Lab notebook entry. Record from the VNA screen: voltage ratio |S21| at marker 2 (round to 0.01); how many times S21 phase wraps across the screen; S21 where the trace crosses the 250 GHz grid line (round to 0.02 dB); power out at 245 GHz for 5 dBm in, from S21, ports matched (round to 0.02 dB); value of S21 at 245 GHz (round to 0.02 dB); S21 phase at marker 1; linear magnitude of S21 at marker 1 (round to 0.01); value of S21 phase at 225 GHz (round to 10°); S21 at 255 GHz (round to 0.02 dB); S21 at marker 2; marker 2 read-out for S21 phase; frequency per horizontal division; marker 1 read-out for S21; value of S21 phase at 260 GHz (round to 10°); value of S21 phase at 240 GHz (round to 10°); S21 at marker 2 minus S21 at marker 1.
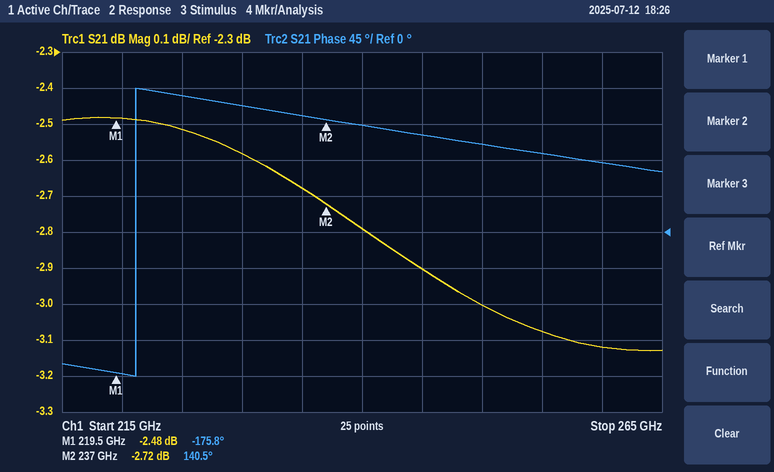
0.73
1
-3.00 dB
2.10 dBm
-2.90 dB
-175.8°
0.75
170°
-3.08 dB
-2.72 dB
140.5°
5 GHz
-2.48 dB
90°
130°
-0.24 dB
